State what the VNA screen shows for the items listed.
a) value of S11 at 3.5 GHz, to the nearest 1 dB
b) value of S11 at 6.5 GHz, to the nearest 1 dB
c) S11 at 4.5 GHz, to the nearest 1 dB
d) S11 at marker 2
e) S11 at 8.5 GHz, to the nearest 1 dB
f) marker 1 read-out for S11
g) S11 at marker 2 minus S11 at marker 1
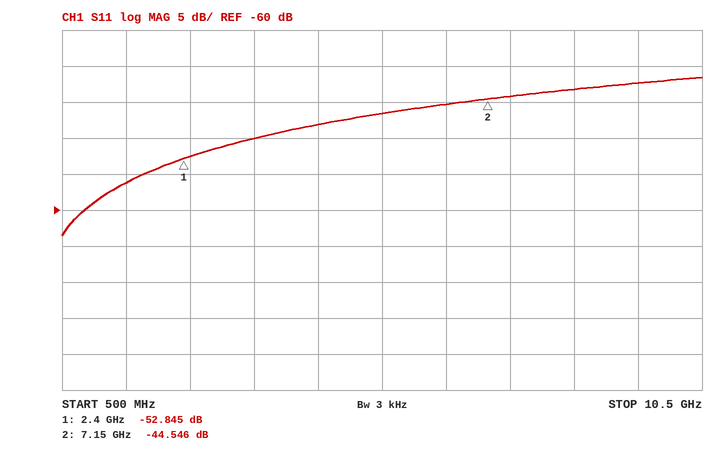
-50 dB
-45 dB
-48 dB
-44.546 dB
-43 dB
-52.845 dB
8.299 dB
